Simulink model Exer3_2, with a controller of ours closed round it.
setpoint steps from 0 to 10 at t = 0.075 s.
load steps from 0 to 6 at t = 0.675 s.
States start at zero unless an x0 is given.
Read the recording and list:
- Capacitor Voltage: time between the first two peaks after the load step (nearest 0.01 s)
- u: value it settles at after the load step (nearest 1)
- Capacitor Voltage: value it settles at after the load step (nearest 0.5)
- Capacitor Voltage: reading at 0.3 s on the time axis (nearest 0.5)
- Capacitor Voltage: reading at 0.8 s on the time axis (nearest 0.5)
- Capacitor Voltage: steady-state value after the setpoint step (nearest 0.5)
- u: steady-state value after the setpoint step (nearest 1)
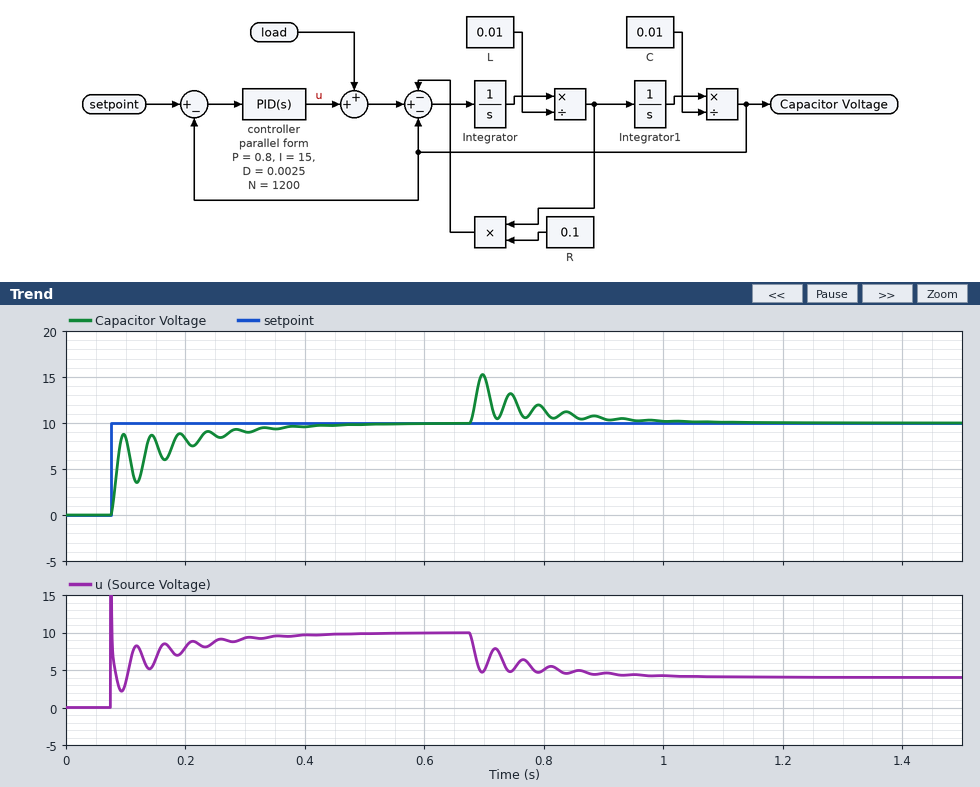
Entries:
0.05 s
4
10.0
9.0
11.5
10.0
10
